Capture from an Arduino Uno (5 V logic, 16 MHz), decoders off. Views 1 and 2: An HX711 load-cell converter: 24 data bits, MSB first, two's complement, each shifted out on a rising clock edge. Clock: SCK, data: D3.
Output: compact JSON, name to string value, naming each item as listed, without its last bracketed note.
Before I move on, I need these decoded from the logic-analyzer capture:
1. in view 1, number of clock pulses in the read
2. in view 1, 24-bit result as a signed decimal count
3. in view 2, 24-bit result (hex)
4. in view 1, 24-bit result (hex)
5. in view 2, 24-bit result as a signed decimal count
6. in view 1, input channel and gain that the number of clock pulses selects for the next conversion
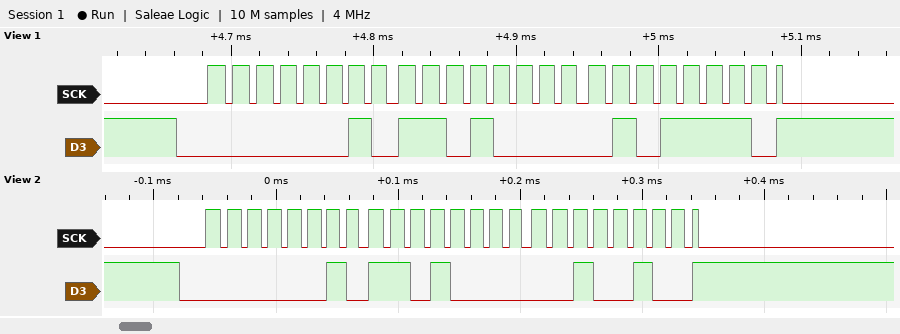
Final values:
{"in view 1, number of clock pulses in the read": "25", "in view 1, 24-bit result as a signed decimal count": "184414", "in view 2, 24-bit result": "0x02D024", "in view 1, 24-bit result": "0x02D05E", "in view 2, 24-bit result as a signed decimal count": "184356", "in view 1, input channel and gain that the number of clock pulses selects for the next conversion": "channel A, gain 128"}
